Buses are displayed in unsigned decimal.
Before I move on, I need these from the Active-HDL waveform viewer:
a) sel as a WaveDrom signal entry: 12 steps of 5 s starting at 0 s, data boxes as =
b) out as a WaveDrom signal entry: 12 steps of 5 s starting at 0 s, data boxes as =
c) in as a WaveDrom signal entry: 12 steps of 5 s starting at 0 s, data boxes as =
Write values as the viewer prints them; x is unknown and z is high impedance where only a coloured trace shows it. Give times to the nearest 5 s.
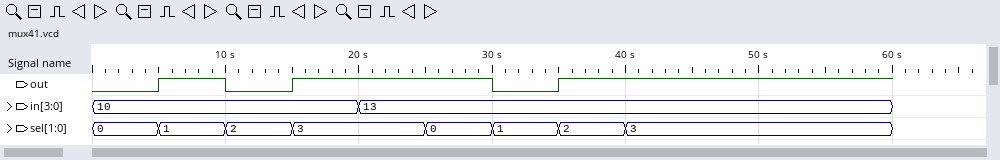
{name: 'sel', wave: '====.====...', data: '0 1 2 3 0 1 2 3'}
{name: 'out', wave: '0101..01....'}
{name: 'in', wave: '=...=.......', data: '10 13'}
